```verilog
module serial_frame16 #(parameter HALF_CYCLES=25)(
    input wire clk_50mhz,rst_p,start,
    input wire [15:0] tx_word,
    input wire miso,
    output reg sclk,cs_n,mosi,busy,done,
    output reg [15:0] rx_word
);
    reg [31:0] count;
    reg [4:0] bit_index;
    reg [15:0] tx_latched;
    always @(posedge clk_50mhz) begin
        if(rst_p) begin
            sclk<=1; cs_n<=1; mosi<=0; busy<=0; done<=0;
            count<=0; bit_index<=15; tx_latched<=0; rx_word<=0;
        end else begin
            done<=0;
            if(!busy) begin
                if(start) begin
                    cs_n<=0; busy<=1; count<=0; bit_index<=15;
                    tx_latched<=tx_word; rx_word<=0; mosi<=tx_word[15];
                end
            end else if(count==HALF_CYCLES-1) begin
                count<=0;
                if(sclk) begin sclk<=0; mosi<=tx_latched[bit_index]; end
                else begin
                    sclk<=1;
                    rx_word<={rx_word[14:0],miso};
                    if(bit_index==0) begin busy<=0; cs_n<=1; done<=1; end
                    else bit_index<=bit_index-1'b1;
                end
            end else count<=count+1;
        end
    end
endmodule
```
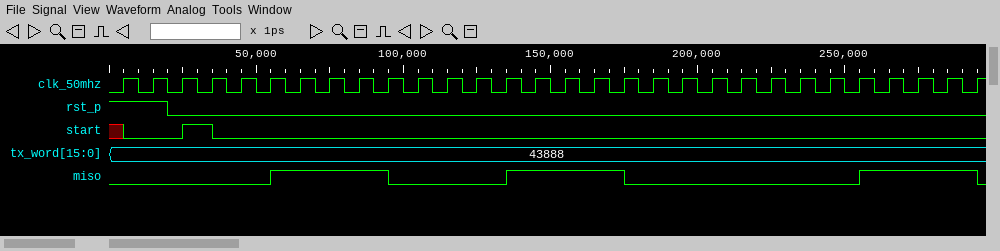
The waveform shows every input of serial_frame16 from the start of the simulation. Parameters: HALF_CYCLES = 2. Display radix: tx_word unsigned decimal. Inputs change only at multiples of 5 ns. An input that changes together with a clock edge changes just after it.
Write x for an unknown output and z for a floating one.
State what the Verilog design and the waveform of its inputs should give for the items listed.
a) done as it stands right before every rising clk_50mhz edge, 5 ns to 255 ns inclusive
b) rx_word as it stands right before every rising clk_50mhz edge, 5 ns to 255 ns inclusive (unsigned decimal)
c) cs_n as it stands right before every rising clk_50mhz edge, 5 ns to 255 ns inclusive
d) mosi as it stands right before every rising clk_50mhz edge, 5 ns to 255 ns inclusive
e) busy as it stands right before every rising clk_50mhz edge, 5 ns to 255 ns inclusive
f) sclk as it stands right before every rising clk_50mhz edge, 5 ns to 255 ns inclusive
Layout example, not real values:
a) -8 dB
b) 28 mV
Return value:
a) x 0 0 0 0 0 0 0 0 0 0 0 0 0 0 0 0 0 0 0 0 0 0 0 0 0
b) x, 0, 0, 0, 0, 0, 0, 0, 1, 1, 1, 1, 2, 2, 2, 2, 5, 5, 5, 5, 10, 10, 10, 10, 20, 20
c) x 1 1 1 0 0 0 0 0 0 0 0 0 0 0 0 0 0 0 0 0 0 0 0 0 0
d) x 0 0 0 1 1 1 1 1 1 0 0 0 0 1 1 1 1 0 0 0 0 1 1 1 1
e) x 0 0 0 1 1 1 1 1 1 1 1 1 1 1 1 1 1 1 1 1 1 1 1 1 1
f) x 1 1 1 1 1 0 0 1 1 0 0 1 1 0 0 1 1 0 0 1 1 0 0 1 1
